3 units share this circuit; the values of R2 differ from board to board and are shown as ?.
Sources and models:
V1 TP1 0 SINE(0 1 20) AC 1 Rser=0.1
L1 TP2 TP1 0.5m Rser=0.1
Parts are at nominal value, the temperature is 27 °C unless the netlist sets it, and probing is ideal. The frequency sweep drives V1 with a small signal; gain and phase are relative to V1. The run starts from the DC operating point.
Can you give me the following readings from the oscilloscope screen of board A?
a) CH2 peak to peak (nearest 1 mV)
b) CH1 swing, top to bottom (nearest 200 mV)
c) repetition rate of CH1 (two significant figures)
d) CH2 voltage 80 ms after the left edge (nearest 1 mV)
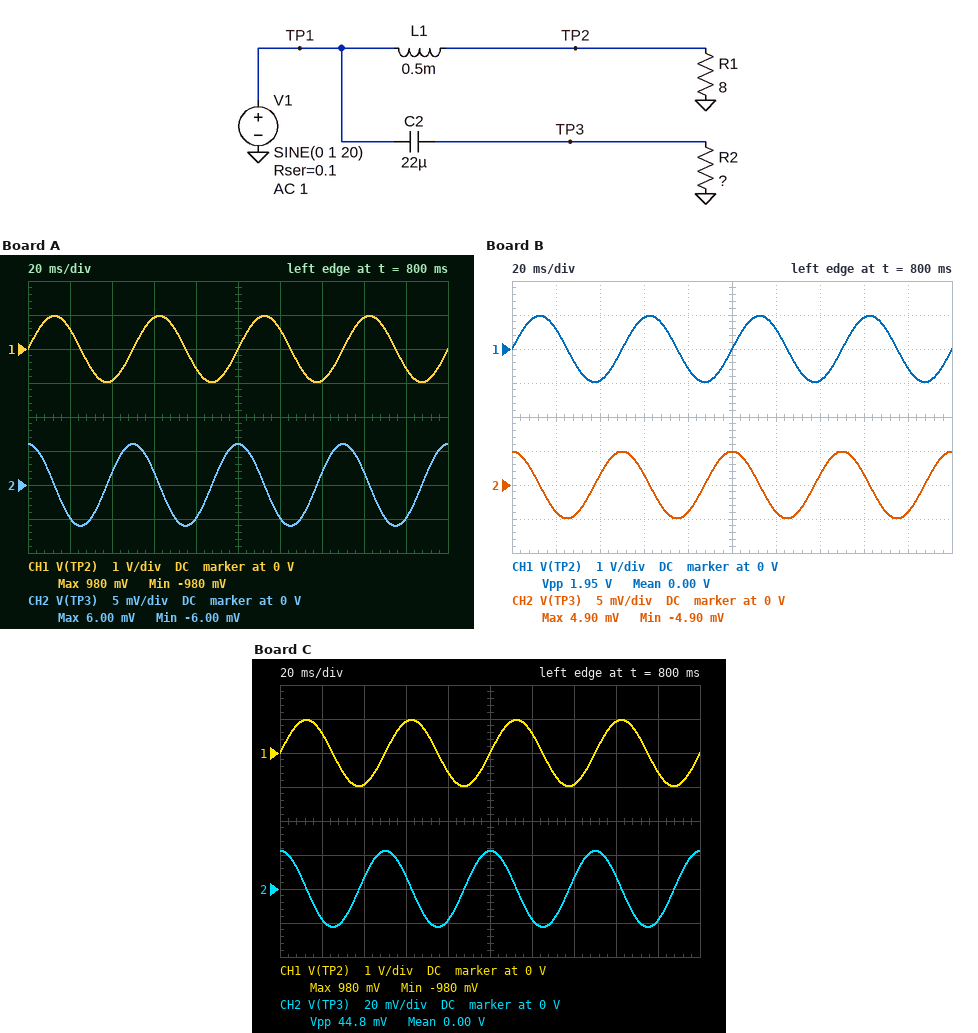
12 mV
2.0 V
20 Hz
-5 mV
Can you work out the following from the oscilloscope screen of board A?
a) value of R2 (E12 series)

2.2 Ω
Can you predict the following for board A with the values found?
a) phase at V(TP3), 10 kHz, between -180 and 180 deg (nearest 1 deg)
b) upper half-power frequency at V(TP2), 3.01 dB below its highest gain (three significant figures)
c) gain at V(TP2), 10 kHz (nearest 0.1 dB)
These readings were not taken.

18 deg
2.52 kHz
-12.5 dB
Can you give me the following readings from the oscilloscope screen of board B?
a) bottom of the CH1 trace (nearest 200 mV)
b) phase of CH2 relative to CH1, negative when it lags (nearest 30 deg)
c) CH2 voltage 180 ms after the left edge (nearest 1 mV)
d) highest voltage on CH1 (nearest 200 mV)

-1.0 V
90 deg
-4 mV
1.0 V
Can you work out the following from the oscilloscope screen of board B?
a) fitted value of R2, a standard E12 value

1.8 Ω
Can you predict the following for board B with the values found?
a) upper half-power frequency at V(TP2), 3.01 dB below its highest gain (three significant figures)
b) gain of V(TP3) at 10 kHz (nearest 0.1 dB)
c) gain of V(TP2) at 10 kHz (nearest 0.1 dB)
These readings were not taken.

2.53 kHz
-1.1 dB
-12.6 dB
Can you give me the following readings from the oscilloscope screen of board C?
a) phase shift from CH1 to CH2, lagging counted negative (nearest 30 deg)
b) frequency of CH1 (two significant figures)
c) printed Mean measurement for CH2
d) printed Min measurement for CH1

90 deg
20 Hz
0.00 V
-980 mV
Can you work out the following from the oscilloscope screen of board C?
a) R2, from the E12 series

8.2 Ω
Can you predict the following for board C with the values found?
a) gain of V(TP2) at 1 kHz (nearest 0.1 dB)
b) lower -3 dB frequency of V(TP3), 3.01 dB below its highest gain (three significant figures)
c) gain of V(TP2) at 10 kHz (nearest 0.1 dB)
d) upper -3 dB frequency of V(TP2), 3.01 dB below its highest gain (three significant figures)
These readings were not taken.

-0.9 dB
891 Hz
-12.3 dB
2.55 kHz
